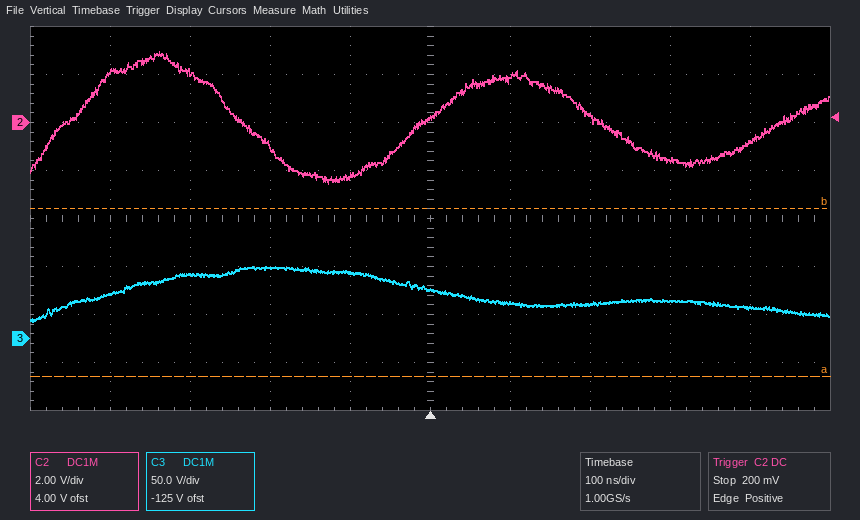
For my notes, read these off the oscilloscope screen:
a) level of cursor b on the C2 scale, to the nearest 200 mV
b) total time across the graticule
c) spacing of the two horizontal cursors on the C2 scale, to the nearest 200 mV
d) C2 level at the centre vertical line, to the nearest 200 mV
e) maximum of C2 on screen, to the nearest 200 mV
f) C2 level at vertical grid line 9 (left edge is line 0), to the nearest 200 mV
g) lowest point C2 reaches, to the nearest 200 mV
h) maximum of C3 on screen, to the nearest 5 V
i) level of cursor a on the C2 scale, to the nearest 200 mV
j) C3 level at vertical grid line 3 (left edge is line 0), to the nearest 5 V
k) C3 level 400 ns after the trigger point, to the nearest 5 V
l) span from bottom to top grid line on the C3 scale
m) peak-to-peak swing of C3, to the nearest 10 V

-3.6 V
1 µs
7.0 V
200 mV
3.0 V
-800 mV
-2.6 V
75 V
-10.6 V
75 V
30 V
400 V
60 V
